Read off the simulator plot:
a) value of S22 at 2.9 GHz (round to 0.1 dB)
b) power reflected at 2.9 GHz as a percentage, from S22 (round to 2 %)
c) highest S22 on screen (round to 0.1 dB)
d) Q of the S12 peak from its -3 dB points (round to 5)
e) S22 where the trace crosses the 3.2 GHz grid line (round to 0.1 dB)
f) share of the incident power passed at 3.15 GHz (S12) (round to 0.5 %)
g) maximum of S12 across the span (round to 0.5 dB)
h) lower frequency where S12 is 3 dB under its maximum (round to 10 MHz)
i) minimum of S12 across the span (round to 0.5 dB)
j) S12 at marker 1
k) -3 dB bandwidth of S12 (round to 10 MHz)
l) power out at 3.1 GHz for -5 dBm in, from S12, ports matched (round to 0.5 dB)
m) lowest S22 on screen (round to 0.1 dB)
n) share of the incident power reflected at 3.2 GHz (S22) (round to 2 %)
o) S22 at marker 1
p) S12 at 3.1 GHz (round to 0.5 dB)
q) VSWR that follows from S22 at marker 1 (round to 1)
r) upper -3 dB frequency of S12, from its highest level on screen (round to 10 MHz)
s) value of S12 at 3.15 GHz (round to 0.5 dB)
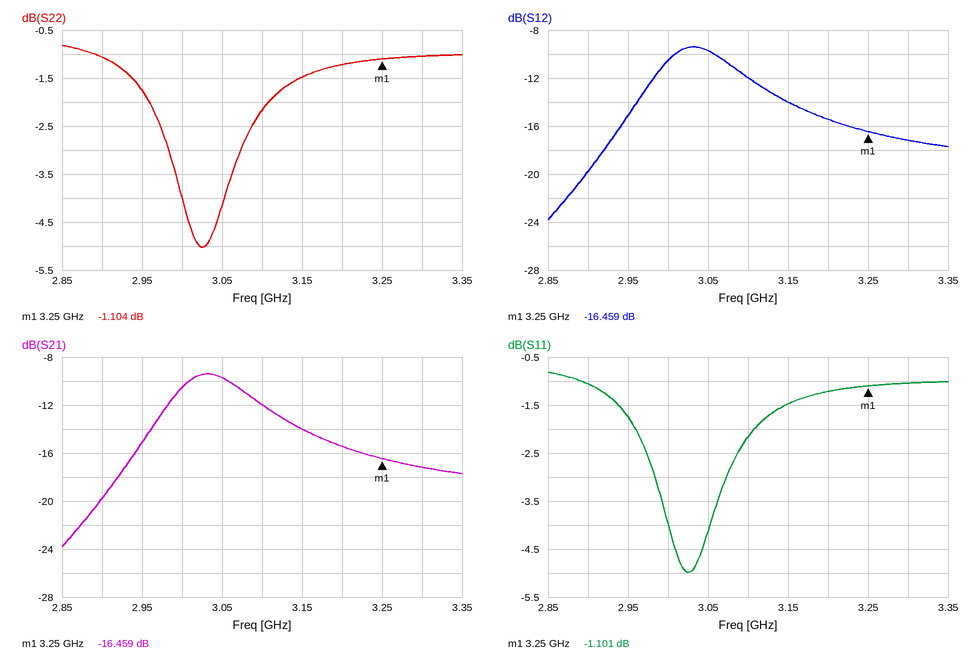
-1.1 dB
78 %
-0.8 dB
25
-1.2 dB
4.0 %
-9.5 dB
2.98 GHz
-24.0 dB
-16.459 dB
130 MHz
-17.0 dBm
-5.0 dB
76 %
-1.104 dB
-12.0 dB
16
3.11 GHz
-14.0 dB
